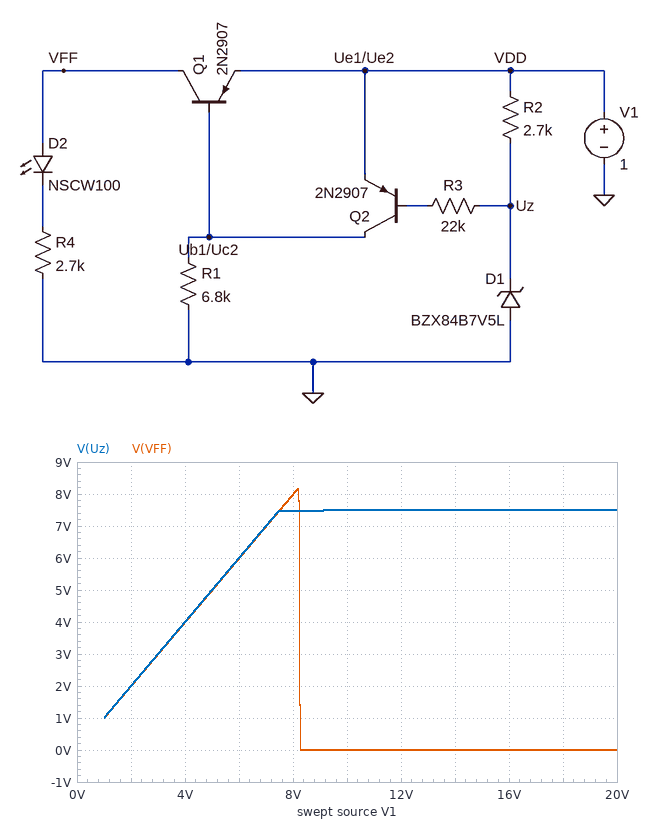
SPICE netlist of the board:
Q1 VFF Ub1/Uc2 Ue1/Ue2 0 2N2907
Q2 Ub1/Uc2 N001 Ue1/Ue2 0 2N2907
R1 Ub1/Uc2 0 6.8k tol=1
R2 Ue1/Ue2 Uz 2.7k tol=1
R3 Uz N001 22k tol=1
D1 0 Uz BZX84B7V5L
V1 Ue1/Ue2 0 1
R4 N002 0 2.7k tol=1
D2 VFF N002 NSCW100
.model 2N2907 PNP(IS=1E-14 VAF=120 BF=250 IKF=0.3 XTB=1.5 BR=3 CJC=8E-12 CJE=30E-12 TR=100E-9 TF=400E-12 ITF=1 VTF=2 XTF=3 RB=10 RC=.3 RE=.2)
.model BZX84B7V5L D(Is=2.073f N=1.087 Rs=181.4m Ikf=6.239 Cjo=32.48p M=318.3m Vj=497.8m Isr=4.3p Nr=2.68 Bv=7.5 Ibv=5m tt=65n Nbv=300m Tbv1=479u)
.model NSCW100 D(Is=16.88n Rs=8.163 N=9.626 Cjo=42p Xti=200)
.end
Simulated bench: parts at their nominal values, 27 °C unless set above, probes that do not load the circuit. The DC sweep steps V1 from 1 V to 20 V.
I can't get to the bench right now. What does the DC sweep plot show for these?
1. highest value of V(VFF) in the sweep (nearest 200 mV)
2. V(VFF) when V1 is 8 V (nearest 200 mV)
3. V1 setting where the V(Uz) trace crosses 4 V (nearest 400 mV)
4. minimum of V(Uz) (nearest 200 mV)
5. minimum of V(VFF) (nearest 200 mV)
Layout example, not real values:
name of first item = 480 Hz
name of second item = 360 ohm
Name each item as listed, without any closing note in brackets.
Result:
highest value of V(VFF) in the sweep = 8.2 V
V(VFF) when V1 is 8 V = 8.0 V
V1 setting where the V(Uz) trace crosses 4 V = 4.0 V
minimum of V(Uz) = 1.0 V
minimum of V(VFF) = 0 V
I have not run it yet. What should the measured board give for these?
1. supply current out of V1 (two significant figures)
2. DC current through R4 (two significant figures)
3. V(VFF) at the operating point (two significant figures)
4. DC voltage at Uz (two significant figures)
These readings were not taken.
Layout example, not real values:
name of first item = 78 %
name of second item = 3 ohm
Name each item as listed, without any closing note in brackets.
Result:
supply current out of V1 = 57 µA
DC current through R4 = 880 nA
V(VFF) at the operating point = 990 mV
DC voltage at Uz = 1.0 V
